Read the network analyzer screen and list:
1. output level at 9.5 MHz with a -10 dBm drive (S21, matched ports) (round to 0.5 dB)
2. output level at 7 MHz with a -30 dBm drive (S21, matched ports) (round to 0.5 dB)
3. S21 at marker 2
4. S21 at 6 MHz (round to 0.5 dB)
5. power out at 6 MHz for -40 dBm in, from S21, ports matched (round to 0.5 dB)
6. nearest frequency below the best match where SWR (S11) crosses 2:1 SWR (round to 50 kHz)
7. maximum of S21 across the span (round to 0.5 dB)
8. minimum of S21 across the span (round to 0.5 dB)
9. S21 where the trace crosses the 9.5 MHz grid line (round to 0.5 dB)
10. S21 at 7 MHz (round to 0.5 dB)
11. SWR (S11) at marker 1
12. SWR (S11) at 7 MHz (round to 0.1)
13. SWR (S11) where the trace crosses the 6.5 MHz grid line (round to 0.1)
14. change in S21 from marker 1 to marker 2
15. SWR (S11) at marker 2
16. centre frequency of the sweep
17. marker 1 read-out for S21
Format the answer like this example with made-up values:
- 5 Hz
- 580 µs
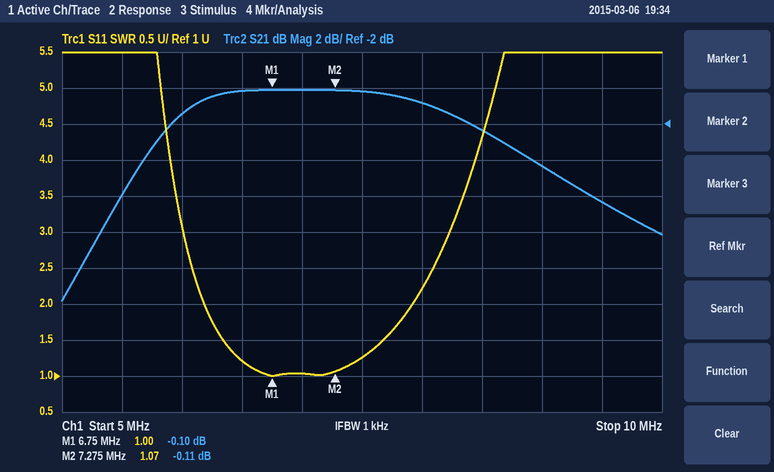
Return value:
- -16.5 dBm
- -30.0 dBm
- -0.11 dB
- -1.5 dB
- -41.5 dBm
- 6.20 MHz
- 0.0 dB
- -12.0 dB
- -6.5 dB
- 0.0 dB
- 1.00
- 1.0
- 1.2
- -0.01 dB
- 1.07
- 7.5 MHz
- -0.10 dB
